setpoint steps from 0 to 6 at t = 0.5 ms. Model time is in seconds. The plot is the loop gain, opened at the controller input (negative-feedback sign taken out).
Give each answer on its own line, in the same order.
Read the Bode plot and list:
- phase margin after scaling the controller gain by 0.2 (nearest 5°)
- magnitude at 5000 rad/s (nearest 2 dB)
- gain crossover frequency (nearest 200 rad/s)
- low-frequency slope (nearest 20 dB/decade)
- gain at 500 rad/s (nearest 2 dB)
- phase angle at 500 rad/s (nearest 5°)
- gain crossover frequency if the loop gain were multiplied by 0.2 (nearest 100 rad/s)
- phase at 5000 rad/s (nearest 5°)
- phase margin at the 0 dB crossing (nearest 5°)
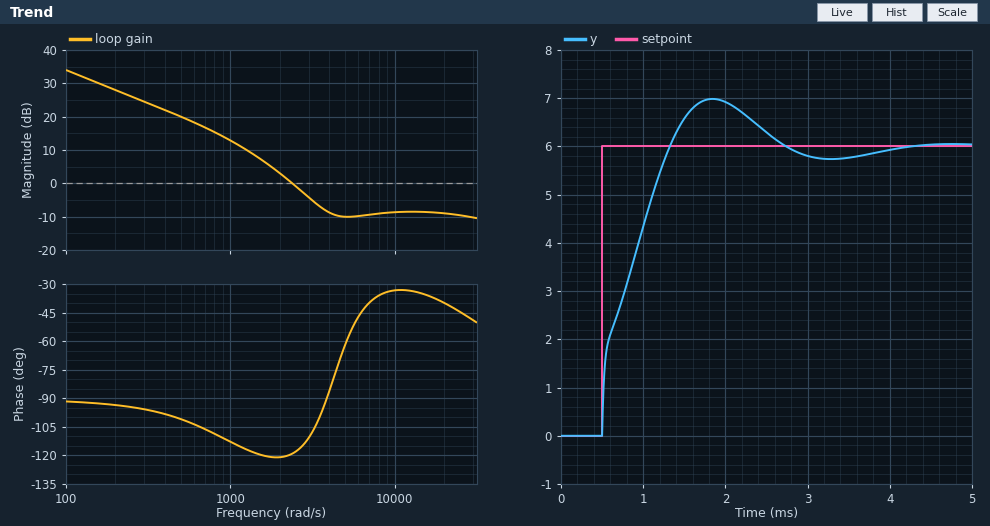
70°
-10 dB
2400 rad/s
-20 dB/decade
20 dB
-100°
900 rad/s
-60°
60°
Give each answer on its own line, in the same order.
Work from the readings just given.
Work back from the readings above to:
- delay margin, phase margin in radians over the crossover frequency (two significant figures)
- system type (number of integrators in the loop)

0.00044 s
1
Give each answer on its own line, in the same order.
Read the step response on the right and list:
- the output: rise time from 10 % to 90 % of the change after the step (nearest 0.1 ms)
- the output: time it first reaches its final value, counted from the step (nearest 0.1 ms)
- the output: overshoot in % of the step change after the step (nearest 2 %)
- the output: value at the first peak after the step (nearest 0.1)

0.7 ms
0.8 ms
16 %
7.0
